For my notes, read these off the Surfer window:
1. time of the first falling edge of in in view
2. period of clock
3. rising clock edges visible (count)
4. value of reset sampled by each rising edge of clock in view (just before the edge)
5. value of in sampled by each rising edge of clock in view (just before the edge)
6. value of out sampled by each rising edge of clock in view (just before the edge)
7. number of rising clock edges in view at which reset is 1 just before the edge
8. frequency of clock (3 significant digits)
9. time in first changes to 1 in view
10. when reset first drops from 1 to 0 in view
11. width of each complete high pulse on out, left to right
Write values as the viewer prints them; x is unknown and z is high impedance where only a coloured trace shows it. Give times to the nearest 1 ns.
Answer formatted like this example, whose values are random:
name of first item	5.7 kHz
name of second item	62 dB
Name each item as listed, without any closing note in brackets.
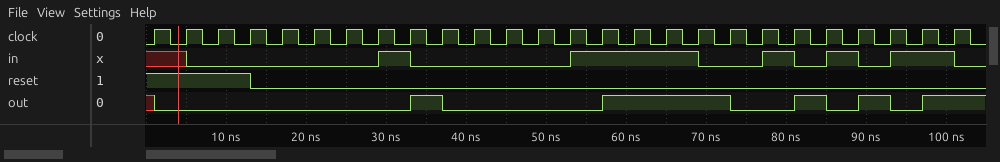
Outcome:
time of the first falling edge of in in view	33 ns
period of clock	4 ns
rising clock edges visible	26
value of reset sampled by each rising edge of clock in view	1 1 1 1 0 0 0 0 0 0 0 0 0 0 0 0 0 0 0 0 0 0 0 0 0 0
value of in sampled by each rising edge of clock in view	x x 0 0 0 0 0 0 1 0 0 0 0 0 1 1 1 1 0 0 1 0 1 0 1 1
value of out sampled by each rising edge of clock in view	x 0 0 0 0 0 0 0 0 1 0 0 0 0 0 1 1 1 1 0 0 1 0 1 0 1
number of rising clock edges in view at which reset is 1 just before the edge	4
frequency of clock	250 MHz
time in first changes to 1 in view	29 ns
when reset first drops from 1 to 0 in view	13 ns
width of each complete high pulse on out, left to right	4 ns, 16 ns, 4 ns, 4 ns
